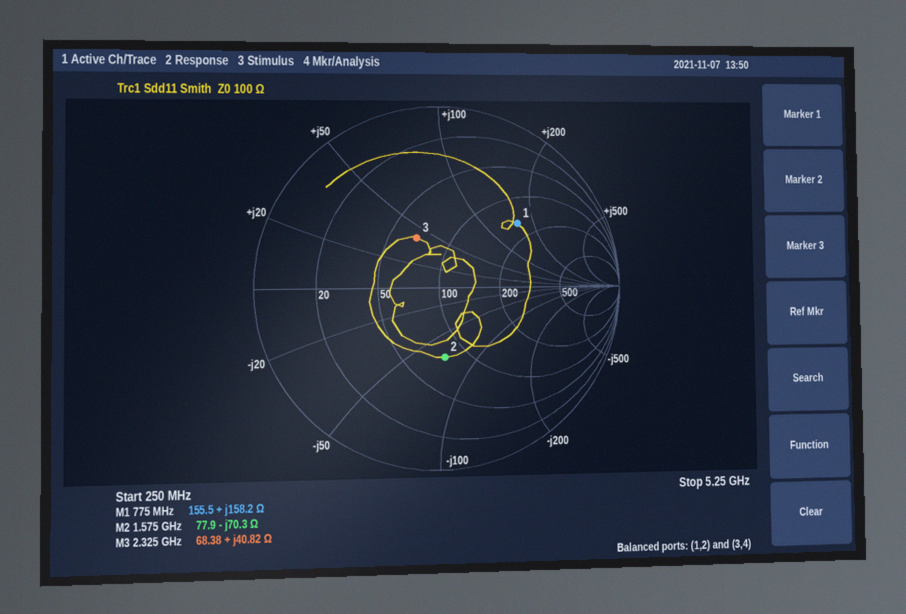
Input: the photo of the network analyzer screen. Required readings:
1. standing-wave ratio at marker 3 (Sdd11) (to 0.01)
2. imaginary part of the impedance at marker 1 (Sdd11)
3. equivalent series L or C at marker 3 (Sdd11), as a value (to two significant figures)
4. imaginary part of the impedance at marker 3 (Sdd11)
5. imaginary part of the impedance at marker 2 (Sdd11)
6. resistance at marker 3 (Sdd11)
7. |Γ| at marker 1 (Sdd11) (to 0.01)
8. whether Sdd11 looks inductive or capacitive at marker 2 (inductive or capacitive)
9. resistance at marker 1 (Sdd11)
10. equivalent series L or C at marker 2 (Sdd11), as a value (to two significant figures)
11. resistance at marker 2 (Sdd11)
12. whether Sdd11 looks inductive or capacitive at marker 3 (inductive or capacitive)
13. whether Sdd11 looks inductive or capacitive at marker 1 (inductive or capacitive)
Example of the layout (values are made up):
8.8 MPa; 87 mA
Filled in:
1.85; +158.2 Ω; 2.8 nH; +40.82 Ω; -70.3 Ω; 68.38 Ω; 0.56; capacitive; 155.5 Ω; 1.4 pF; 77.9 Ω; inductive; inductive
